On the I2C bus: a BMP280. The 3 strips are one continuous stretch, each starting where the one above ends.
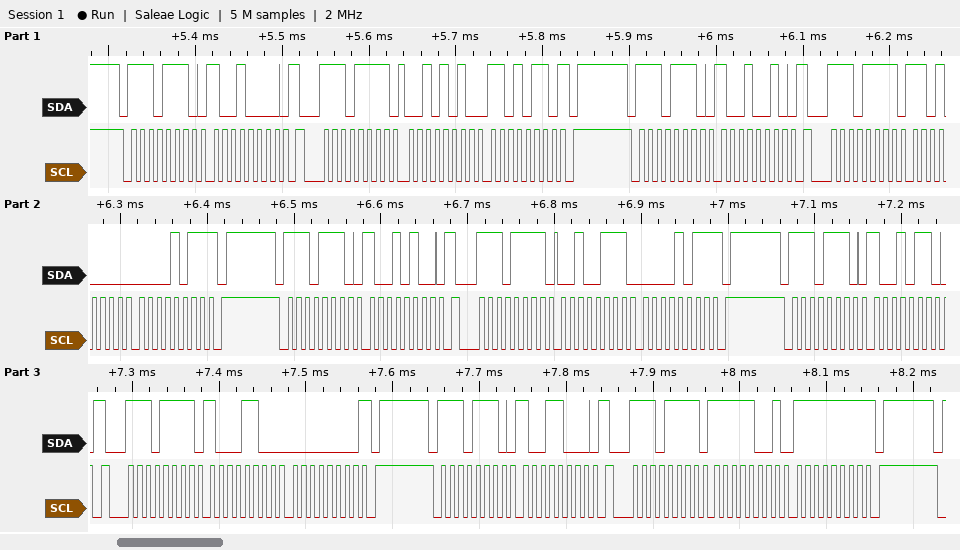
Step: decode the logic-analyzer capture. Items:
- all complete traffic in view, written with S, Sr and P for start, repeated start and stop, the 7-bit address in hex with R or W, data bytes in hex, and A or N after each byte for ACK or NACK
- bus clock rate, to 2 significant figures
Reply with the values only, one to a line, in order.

S 77W A 90 A Sr 77R A 2A A D6 N P S 77W A 92 A Sr 77R A D0 A 0B N P S 77W A 94 A Sr 77R A 27 A 0B N P S 77W A 96 A Sr 77R A 8C A 00 N P S 77W A 98 A Sr 77R A F9 A FF N P
100 kHz
